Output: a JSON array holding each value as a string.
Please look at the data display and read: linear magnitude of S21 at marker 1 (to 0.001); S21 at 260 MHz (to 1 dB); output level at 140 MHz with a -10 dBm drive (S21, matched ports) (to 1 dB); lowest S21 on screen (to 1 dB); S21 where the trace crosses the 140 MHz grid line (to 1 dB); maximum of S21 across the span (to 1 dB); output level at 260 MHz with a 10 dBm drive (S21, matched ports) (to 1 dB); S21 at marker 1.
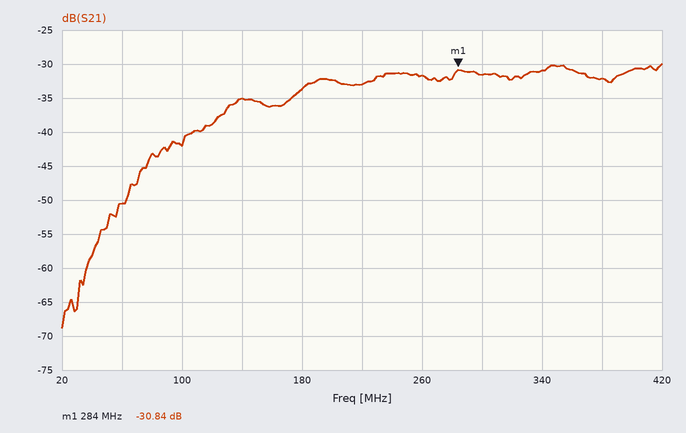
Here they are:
["0.029", "-32 dB", "-45 dBm", "-69 dB", "-35 dB", "-30 dB", "-22 dBm", "-30.84 dB"]
